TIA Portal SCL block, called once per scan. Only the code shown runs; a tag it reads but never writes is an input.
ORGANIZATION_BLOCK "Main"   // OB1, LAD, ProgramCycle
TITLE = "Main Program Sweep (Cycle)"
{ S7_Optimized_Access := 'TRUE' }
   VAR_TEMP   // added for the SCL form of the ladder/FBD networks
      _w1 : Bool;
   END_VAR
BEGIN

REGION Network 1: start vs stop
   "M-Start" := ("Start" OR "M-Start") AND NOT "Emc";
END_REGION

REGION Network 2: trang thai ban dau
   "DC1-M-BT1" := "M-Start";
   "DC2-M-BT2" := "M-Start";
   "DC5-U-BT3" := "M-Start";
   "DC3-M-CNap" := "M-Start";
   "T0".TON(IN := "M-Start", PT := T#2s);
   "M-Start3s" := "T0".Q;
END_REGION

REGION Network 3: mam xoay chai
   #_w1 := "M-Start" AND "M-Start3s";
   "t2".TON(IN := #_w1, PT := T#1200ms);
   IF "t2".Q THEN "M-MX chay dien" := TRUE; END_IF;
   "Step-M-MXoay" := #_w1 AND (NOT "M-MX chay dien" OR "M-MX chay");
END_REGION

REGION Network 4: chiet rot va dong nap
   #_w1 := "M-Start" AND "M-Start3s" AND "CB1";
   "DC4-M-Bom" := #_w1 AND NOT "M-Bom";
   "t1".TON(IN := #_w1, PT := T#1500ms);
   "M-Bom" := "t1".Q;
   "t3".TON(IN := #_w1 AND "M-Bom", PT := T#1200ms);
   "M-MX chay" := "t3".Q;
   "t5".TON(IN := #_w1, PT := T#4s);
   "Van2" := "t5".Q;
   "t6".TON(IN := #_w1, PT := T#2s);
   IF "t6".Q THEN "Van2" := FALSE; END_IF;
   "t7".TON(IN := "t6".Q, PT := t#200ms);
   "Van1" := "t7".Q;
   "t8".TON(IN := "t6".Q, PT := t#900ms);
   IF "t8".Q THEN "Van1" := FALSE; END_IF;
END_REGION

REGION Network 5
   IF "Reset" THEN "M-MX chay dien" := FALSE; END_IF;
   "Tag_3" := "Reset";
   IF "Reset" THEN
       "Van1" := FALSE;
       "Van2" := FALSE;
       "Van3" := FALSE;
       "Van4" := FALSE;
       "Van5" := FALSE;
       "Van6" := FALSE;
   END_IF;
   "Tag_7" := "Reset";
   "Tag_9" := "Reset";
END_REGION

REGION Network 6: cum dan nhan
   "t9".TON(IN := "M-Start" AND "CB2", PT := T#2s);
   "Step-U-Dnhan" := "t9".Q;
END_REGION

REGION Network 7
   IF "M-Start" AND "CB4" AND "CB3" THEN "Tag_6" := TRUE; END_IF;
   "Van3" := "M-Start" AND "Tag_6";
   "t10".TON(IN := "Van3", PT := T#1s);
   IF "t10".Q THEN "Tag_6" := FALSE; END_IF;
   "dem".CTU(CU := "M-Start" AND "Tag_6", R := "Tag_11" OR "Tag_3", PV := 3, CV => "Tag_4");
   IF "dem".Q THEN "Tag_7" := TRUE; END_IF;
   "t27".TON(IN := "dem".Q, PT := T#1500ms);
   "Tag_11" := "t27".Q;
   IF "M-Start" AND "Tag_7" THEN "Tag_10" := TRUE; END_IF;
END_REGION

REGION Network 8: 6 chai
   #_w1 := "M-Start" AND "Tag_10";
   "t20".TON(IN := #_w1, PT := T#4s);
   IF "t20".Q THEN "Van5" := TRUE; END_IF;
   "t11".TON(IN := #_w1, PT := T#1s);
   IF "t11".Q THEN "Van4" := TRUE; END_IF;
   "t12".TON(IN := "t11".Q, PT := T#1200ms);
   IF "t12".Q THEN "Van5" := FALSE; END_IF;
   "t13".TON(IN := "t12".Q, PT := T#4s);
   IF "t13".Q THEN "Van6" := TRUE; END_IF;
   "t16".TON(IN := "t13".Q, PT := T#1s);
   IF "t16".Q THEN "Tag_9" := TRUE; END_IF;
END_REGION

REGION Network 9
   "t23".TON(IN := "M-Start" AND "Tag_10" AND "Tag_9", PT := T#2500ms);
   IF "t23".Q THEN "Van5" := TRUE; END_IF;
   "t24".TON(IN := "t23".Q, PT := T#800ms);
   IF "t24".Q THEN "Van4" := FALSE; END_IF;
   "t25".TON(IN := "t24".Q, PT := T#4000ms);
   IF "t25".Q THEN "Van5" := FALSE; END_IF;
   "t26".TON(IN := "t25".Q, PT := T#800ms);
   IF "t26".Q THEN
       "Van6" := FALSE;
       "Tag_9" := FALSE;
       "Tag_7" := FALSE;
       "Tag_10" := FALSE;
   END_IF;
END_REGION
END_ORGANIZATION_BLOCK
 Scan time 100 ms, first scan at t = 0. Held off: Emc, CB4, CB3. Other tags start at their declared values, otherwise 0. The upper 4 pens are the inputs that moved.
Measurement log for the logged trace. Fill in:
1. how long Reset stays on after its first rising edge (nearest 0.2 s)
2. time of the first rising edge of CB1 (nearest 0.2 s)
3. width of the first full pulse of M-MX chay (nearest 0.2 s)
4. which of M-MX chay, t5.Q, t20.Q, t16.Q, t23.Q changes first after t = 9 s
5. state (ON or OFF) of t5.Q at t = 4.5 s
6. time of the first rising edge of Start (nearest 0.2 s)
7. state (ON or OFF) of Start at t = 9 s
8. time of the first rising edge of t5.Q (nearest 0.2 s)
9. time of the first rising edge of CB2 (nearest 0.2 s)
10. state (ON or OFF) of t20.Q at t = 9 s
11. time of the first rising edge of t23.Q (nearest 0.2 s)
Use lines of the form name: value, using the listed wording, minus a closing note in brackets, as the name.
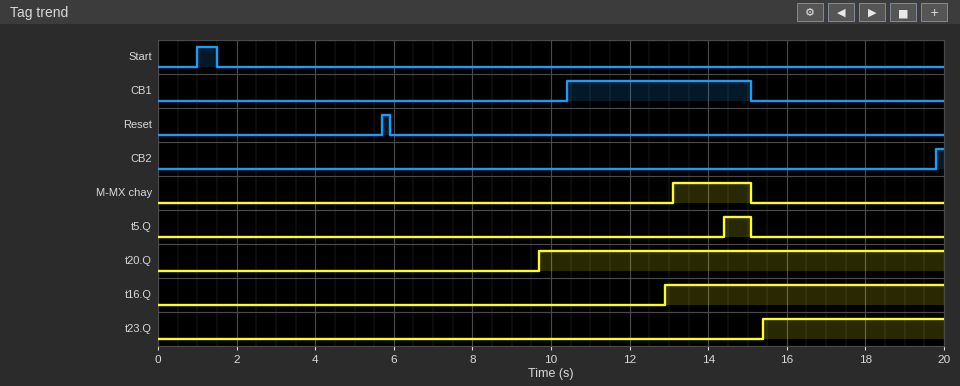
how long Reset stays on after its first rising edge: 0.2 s
time of the first rising edge of CB1: 10.4 s
width of the first full pulse of M-MX chay: 2.0 s
which of M-MX chay, t5.Q, t20.Q, t16.Q, t23.Q changes first after t = 9 s: t20.Q
state (ON or OFF) of t5.Q at t = 4.5 s: OFF
time of the first rising edge of Start: 1.0 s
state (ON or OFF) of Start at t = 9 s: OFF
time of the first rising edge of t5.Q: 14.4 s
time of the first rising edge of CB2: 19.8 s
state (ON or OFF) of t20.Q at t = 9 s: OFF
time of the first rising edge of t23.Q: 15.4 s
